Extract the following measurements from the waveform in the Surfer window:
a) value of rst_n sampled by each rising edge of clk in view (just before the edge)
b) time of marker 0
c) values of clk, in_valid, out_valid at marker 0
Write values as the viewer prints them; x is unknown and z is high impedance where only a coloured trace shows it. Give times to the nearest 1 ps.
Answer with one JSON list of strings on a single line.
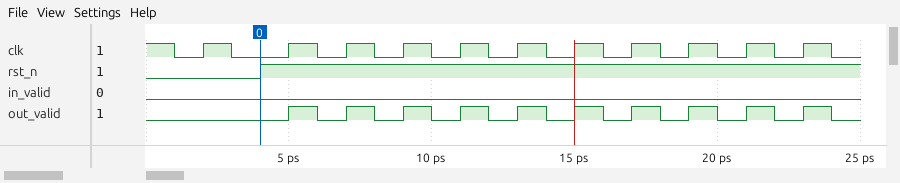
["0 1 1 1 1 1 1 1 1 1 1", "4 ps", "clk=0, in_valid=0, out_valid=0"]
